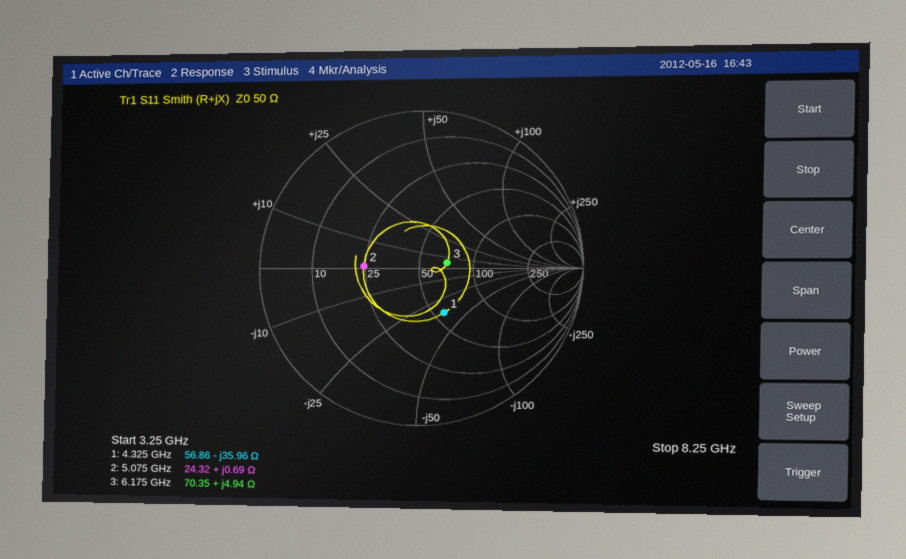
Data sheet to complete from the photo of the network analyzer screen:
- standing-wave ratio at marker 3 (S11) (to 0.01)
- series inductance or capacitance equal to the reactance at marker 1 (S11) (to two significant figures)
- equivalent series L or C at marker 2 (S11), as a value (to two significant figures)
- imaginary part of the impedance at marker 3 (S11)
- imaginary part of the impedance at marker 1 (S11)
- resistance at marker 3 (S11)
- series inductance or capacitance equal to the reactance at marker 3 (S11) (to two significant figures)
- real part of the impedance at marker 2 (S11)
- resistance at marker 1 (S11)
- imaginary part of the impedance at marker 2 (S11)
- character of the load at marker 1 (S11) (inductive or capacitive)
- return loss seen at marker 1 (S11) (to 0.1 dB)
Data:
1.42
1.0 pF
22 pH
+4.94 Ω
-35.96 Ω
70.35 Ω
130 pH
24.32 Ω
56.86 Ω
+0.69 Ω
capacitive
9.8 dB
